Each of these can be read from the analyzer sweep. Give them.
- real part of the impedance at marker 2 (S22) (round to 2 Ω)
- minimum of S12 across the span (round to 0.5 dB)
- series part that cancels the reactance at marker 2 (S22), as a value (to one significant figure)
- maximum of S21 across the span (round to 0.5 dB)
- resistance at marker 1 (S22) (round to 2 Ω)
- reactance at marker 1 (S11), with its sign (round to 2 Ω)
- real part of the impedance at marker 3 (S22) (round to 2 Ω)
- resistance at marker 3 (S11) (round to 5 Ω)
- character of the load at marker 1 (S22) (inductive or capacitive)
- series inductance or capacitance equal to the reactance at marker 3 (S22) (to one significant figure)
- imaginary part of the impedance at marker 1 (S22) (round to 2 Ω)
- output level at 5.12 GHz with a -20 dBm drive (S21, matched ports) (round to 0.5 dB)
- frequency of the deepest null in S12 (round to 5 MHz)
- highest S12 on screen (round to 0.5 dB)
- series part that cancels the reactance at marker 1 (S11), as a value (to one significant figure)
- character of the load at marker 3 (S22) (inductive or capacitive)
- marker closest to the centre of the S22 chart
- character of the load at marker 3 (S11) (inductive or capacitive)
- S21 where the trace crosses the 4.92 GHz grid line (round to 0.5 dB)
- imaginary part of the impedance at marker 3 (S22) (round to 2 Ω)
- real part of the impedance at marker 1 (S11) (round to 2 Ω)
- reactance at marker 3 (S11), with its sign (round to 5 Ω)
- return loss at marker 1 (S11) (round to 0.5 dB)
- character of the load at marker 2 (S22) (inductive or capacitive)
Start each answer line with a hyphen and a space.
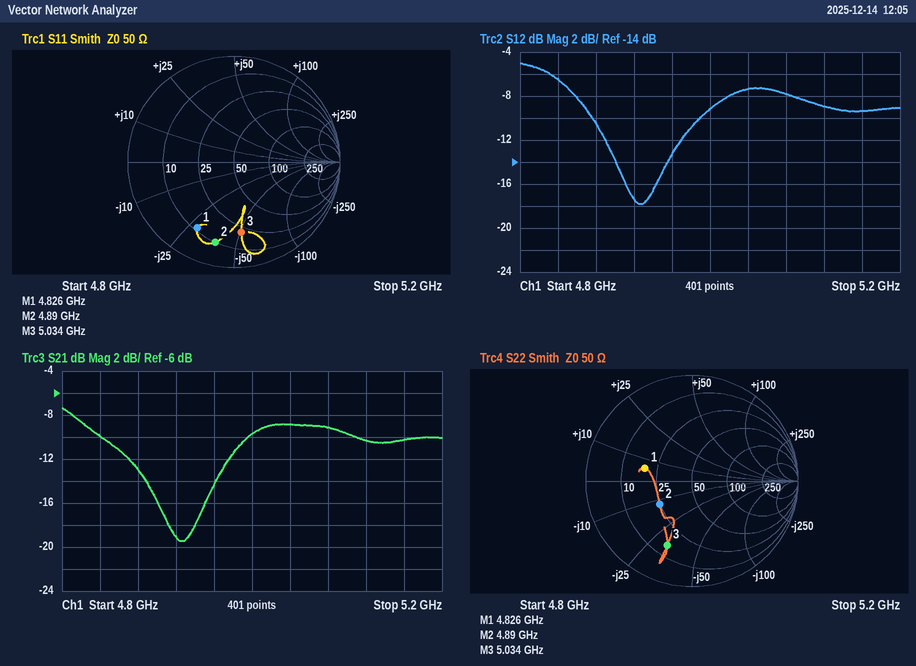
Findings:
- 24 Ω
- -18.0 dB
- 400 pH
- -7.5 dB
- 18 Ω
- -28 Ω
- 16 Ω
- 20 Ω
- inductive
- 1.0 pF
- +6 Ω
- -30.5 dBm
- 4.925 GHz
- -5.0 dB
- 900 pH
- capacitive
- marker 2
- capacitive
- -19.0 dB
- -32 Ω
- 12 Ω
- -50 Ω
- 3.0 dB
- capacitive
